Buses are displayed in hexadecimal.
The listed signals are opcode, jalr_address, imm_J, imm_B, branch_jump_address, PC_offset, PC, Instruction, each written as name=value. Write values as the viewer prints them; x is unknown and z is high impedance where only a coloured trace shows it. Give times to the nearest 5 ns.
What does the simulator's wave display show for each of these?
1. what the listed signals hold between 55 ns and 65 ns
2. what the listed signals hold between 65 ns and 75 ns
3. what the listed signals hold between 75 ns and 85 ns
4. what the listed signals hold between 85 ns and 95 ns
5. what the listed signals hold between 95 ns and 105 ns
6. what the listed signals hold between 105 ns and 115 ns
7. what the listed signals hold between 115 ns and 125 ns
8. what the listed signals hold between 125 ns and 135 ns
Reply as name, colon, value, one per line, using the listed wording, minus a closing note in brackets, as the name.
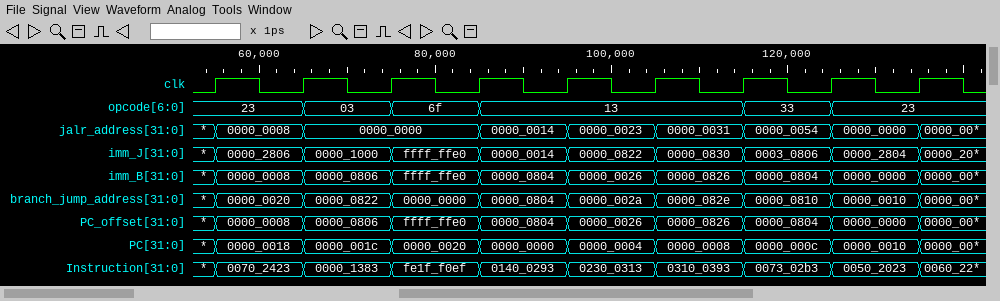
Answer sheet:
what the listed signals hold between 55 ns and 65 ns: opcode=23, jalr_address=0000_0008, imm_J=0000_2806, imm_B=0000_0008, branch_jump_address=0000_0020, PC_offset=0000_0008, PC=0000_0018, Instruction=0070_2423
what the listed signals hold between 65 ns and 75 ns: opcode=03, jalr_address=0000_0000, imm_J=0000_1000, imm_B=0000_0806, branch_jump_address=0000_0822, PC_offset=0000_0806, PC=0000_001c, Instruction=0000_1383
what the listed signals hold between 75 ns and 85 ns: opcode=6f, jalr_address=0000_0000, imm_J=ffff_ffe0, imm_B=ffff_ffe0, branch_jump_address=0000_0000, PC_offset=ffff_ffe0, PC=0000_0020, Instruction=fe1f_f0ef
what the listed signals hold between 85 ns and 95 ns: opcode=13, jalr_address=0000_0014, imm_J=0000_0014, imm_B=0000_0804, branch_jump_address=0000_0804, PC_offset=0000_0804, PC=0000_0000, Instruction=0140_0293
what the listed signals hold between 95 ns and 105 ns: opcode=13, jalr_address=0000_0023, imm_J=0000_0822, imm_B=0000_0026, branch_jump_address=0000_002a, PC_offset=0000_0026, PC=0000_0004, Instruction=0230_0313
what the listed signals hold between 105 ns and 115 ns: opcode=13, jalr_address=0000_0031, imm_J=0000_0830, imm_B=0000_0826, branch_jump_address=0000_082e, PC_offset=0000_0826, PC=0000_0008, Instruction=0310_0393
what the listed signals hold between 115 ns and 125 ns: opcode=33, jalr_address=0000_0054, imm_J=0003_0806, imm_B=0000_0804, branch_jump_address=0000_0810, PC_offset=0000_0804, PC=0000_000c, Instruction=0073_02b3
what the listed signals hold between 125 ns and 135 ns: opcode=23, jalr_address=0000_0000, imm_J=0000_2804, imm_B=0000_0000, branch_jump_address=0000_0010, PC_offset=0000_0000, PC=0000_0010, Instruction=0050_2023
